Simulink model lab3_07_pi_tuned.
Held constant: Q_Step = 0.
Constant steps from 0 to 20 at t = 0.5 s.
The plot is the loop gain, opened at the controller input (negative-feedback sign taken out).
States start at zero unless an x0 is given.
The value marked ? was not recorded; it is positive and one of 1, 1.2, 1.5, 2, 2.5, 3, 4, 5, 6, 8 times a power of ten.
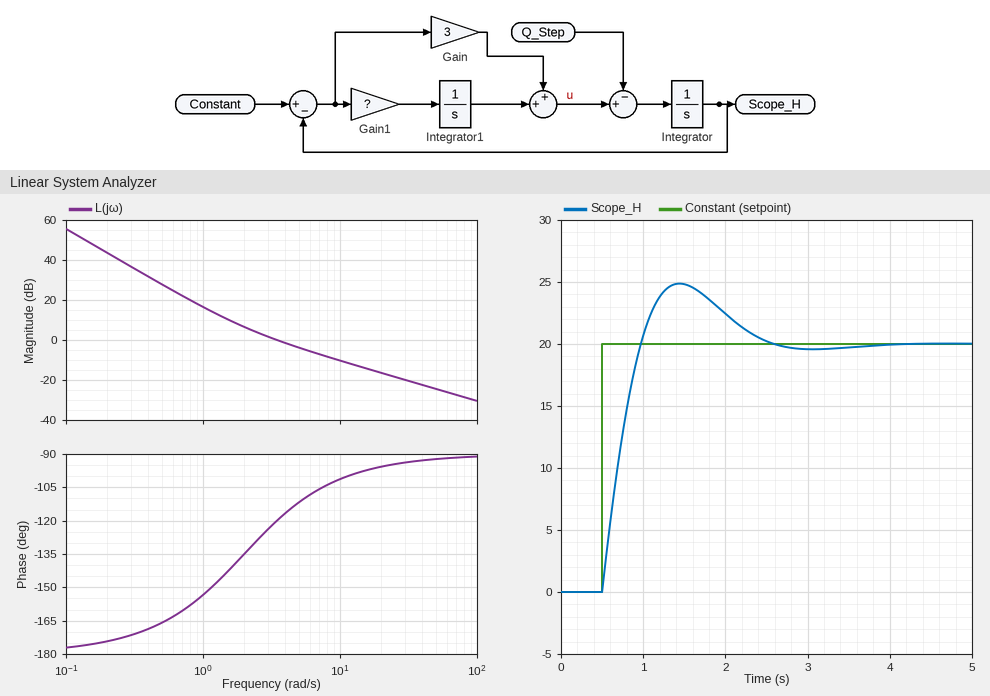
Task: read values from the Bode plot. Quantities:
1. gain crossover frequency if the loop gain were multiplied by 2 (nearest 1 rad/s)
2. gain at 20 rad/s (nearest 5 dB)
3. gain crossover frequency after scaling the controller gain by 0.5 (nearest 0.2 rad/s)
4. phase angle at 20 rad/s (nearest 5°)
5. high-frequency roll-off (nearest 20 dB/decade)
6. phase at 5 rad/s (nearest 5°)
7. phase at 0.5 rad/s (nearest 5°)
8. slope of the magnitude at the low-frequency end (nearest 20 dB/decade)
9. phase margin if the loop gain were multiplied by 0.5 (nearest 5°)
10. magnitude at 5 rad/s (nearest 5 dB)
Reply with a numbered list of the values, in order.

1. 6 rad/s
2. -15 dB
3. 2.0 rad/s
4. -95°
5. -20 dB/decade
6. -110°
7. -165°
8. -40 dB/decade
9. 45°
10. -5 dB
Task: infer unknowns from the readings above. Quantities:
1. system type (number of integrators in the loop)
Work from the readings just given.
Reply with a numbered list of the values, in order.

1. 2
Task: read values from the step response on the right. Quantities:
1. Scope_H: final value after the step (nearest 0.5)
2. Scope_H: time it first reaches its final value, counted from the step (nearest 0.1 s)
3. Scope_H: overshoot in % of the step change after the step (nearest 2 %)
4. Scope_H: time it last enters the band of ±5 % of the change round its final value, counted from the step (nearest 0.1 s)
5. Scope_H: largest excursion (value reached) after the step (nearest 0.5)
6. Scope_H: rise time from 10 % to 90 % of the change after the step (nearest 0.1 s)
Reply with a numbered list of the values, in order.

1. 20.0
2. 0.5 s
3. 24 %
4. 1.8 s
5. 25.0
6. 0.4 s
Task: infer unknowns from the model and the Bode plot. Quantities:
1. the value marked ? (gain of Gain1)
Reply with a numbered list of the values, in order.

1. 6
